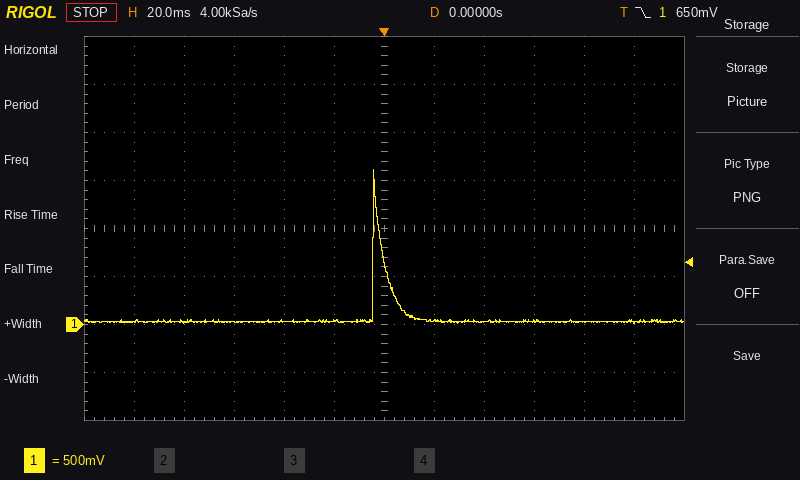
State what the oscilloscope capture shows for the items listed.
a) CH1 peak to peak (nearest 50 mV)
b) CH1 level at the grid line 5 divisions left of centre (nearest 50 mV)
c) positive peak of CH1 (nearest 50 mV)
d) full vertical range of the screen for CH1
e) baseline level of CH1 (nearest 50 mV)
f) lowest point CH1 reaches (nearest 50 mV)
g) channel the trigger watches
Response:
1.60 V
50 mV
1.60 V
4 V
50 mV
0 mV
CH1
